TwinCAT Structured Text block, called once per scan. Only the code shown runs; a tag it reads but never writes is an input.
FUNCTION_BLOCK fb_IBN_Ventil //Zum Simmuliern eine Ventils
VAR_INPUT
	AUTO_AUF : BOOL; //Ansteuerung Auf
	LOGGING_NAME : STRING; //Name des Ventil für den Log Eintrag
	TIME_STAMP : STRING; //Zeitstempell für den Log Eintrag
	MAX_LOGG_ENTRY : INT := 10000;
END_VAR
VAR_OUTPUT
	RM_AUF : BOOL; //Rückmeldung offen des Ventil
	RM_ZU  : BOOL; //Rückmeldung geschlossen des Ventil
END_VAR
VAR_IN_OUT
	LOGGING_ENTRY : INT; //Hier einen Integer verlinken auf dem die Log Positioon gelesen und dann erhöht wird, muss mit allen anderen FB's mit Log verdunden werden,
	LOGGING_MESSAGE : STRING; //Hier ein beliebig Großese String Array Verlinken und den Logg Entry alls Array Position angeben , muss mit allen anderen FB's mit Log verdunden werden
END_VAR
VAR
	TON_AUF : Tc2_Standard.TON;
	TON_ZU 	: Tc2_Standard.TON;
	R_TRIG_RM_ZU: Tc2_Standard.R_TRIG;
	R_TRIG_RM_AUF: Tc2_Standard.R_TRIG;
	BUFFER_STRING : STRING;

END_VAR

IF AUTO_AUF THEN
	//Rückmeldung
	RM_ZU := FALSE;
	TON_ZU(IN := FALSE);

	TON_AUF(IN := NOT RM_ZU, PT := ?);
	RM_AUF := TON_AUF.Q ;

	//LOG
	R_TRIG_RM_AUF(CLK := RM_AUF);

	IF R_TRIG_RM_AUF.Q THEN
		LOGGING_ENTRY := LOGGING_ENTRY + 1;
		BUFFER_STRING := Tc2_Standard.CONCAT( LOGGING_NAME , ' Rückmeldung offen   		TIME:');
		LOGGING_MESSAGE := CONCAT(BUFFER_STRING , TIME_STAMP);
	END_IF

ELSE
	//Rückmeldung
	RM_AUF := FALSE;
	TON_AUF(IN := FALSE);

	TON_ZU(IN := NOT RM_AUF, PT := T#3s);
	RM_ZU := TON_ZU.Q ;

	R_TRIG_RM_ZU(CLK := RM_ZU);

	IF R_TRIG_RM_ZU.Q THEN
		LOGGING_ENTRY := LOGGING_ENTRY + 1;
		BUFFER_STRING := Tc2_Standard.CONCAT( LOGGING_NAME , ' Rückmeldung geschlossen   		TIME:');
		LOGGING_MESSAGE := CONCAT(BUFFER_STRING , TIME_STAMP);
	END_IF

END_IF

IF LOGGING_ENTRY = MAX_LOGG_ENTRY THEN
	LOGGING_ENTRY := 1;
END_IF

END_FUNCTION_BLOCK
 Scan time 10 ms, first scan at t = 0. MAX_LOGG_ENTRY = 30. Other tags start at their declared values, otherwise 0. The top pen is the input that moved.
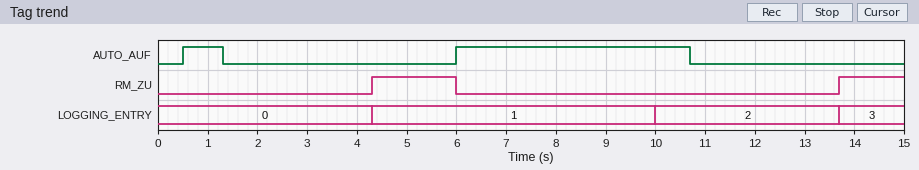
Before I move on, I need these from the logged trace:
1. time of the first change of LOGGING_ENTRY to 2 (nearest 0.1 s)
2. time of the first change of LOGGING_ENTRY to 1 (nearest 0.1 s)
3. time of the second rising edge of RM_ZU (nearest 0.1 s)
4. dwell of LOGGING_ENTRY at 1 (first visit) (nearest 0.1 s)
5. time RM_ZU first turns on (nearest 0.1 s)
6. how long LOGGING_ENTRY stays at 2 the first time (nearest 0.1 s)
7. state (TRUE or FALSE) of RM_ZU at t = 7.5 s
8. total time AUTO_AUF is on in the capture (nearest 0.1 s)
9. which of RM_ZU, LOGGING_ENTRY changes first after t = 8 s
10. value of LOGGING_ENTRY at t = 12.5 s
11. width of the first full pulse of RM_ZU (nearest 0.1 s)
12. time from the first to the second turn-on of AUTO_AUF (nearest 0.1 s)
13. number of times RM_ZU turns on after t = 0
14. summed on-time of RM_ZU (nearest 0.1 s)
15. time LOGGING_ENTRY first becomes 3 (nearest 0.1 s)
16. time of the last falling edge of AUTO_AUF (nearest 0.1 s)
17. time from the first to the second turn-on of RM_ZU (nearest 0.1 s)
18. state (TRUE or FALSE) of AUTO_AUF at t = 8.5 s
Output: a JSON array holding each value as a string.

["10.0 s", "4.3 s", "13.7 s", "5.7 s", "4.3 s", "3.7 s", "FALSE", "5.5 s", "LOGGING_ENTRY", "2", "1.7 s", "5.5 s", "2", "3.0 s", "13.7 s", "10.7 s", "9.4 s", "TRUE"]
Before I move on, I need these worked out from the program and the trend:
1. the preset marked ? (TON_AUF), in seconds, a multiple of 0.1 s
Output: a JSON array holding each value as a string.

["4.0 s"]
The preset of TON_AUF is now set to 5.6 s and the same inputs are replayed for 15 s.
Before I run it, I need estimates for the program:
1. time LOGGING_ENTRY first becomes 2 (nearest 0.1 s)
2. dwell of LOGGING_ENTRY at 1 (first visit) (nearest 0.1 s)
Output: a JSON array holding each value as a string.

["13.7 s", "9.4 s"]
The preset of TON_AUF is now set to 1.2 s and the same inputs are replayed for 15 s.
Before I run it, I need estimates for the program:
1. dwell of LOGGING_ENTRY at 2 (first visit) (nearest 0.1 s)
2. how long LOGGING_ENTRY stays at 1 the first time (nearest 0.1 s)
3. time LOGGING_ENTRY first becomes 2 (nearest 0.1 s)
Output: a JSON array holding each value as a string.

["6.5 s", "2.9 s", "7.2 s"]
